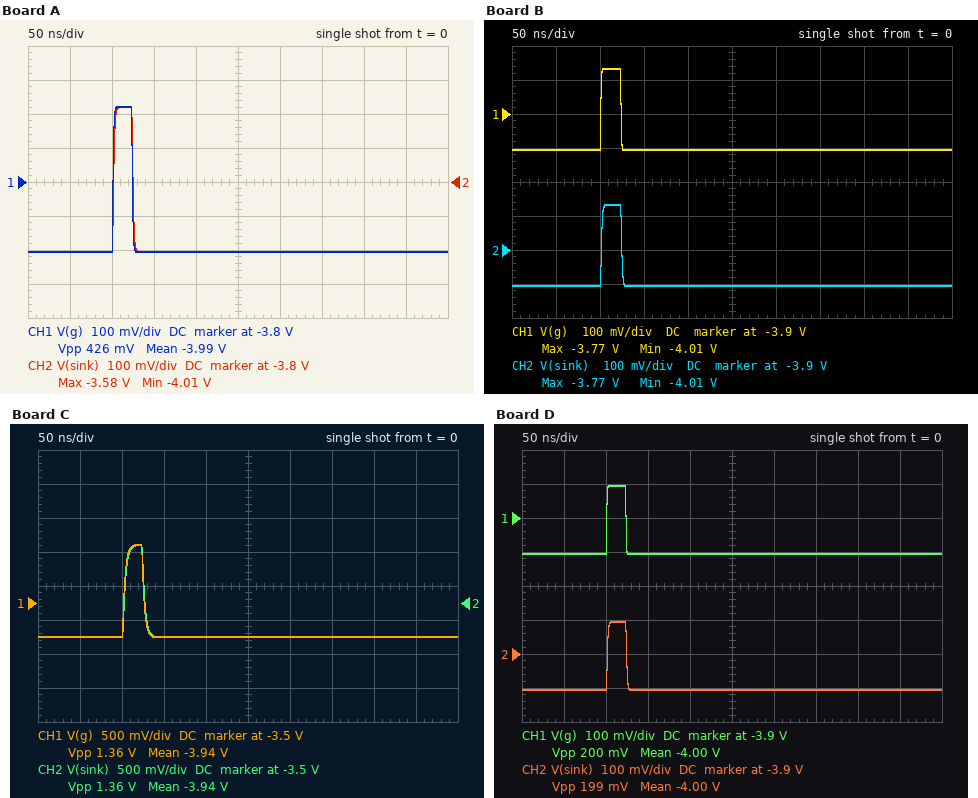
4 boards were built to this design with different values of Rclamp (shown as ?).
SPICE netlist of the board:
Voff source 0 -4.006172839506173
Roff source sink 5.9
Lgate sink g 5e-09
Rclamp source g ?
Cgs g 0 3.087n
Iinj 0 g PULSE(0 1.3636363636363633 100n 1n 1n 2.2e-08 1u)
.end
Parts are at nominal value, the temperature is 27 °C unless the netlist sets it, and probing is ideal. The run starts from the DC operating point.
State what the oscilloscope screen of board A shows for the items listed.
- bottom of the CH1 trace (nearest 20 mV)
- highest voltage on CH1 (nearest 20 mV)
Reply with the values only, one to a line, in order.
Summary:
-4.00 V
-3.58 V
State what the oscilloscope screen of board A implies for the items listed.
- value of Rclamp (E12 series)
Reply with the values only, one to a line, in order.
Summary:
0.33 Ω
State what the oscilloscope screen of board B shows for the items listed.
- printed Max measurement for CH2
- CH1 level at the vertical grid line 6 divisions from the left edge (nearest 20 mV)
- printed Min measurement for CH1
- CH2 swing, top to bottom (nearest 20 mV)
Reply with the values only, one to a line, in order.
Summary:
-3.77 V
-4.00 V
-4.01 V
240 mV
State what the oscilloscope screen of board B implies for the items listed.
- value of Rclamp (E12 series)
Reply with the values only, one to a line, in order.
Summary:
0.18 Ω
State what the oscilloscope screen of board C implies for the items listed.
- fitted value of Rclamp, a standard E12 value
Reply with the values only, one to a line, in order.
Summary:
1.2 Ω
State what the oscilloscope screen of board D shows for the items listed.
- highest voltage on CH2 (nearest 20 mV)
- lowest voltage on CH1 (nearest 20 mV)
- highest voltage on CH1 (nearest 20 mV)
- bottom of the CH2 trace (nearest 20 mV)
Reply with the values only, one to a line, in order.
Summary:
-3.80 V
-4.00 V
-3.80 V
-4.00 V
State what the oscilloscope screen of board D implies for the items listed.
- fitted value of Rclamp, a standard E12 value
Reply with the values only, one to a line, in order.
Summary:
0.15 Ω
